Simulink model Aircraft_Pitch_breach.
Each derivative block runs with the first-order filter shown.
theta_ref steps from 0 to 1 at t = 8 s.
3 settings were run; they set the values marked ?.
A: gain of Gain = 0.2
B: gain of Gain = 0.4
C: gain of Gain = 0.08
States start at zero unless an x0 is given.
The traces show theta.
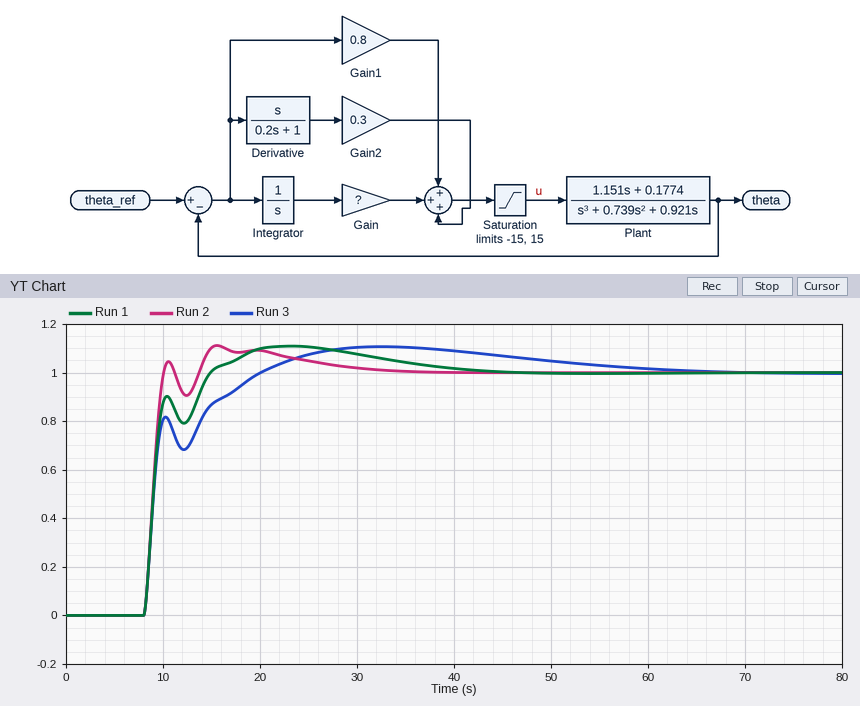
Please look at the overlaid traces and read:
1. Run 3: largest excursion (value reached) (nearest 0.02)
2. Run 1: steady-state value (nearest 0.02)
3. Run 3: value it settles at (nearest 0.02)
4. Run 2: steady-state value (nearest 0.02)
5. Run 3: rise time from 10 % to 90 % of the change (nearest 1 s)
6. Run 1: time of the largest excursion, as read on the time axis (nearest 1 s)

1.10
1.00
1.00
1.00
8 s
23 s
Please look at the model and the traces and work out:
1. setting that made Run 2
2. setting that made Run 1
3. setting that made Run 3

B
A
C
